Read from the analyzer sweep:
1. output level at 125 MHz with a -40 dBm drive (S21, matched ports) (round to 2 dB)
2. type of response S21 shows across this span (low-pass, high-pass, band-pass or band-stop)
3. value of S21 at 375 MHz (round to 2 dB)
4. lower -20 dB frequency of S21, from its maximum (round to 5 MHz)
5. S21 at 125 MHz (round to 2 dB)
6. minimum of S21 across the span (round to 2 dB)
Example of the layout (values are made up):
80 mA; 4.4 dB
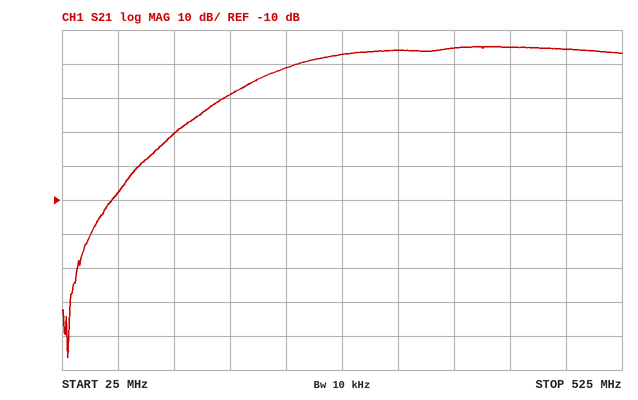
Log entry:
-30 dBm; high-pass; 34 dB; 150 MHz; 10 dB; -56 dB
